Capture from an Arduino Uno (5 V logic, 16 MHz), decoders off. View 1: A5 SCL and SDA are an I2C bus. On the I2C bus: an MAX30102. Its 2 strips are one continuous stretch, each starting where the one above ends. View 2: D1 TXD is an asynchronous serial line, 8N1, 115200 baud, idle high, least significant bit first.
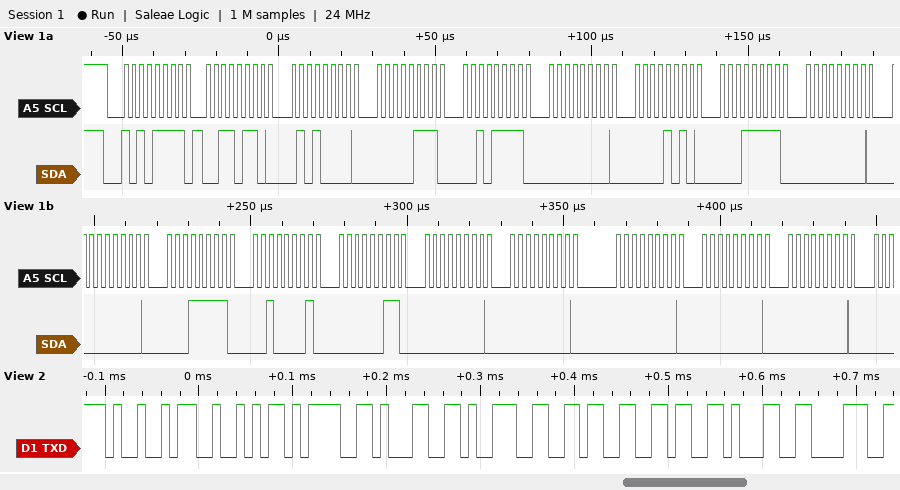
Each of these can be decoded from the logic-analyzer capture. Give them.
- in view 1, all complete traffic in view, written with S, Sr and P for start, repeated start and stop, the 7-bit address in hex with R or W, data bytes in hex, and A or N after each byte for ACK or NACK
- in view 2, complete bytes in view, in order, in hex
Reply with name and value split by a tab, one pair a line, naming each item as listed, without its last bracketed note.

in view 1, all complete traffic in view, written with S, Sr and P for start, repeated start and stop, the 7-bit address in hex with R or W, data bytes in hex, and A or N after each byte for ACK or NACK	S 57R A 36 A 50 A 07 A 2F A 00 A 0A A 1F A 00 A 00 A 1F A 21 A 03 A 00 A 00 A 00 A 00 A 00 A
in view 2, complete bytes in view, in order, in hex	49 52 3D 31 39 36 36 31 38
